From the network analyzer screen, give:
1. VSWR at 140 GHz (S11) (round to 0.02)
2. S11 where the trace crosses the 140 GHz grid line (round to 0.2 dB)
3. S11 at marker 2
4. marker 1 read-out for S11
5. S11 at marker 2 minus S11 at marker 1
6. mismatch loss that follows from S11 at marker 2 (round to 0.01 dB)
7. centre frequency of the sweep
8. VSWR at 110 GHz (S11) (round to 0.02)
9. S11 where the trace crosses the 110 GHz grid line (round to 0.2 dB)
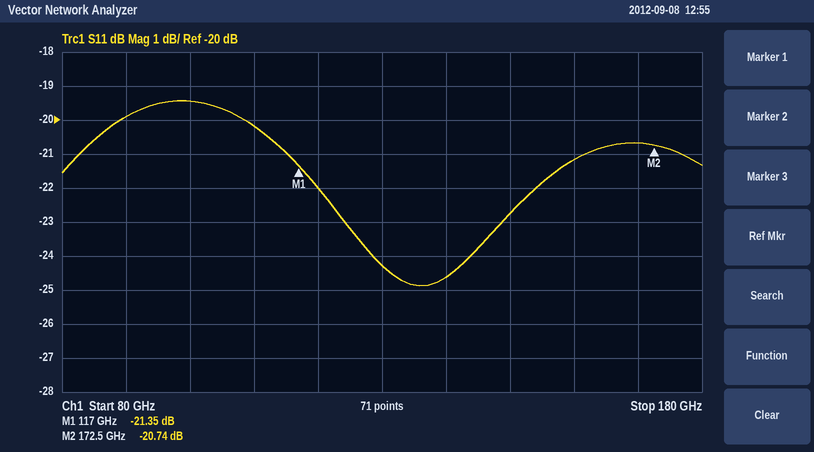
1.12
-24.6 dB
-20.74 dB
-21.35 dB
0.61 dB
0.04 dB
130 GHz
1.22
-20.2 dB
